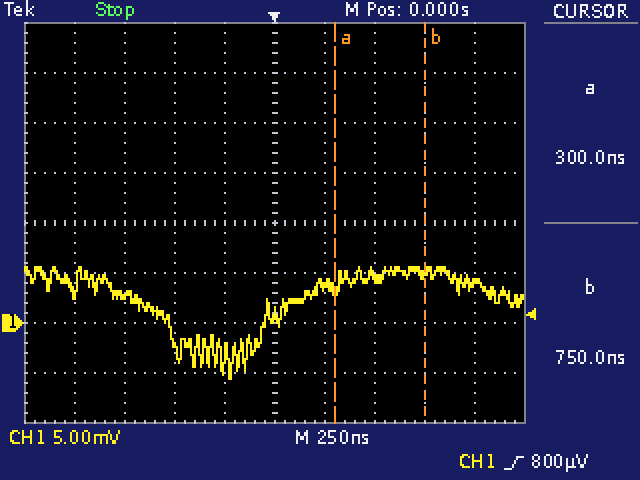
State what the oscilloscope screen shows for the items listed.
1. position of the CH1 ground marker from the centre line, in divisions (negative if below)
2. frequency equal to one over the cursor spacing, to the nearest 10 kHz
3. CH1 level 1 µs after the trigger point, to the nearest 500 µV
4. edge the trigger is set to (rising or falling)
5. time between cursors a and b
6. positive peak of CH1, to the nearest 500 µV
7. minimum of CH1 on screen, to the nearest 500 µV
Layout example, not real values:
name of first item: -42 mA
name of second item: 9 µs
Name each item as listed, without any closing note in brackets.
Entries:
position of the CH1 ground marker from the centre line, in divisions: -2.0 div
frequency equal to one over the cursor spacing, to the nearest 10 kHz: 2.22 MHz
CH1 level 1 µs after the trigger point, to the nearest 500 µV: 4.0 mV
edge the trigger is set to: rising
time between cursors a and b: 450 ns
positive peak of CH1, to the nearest 500 µV: 5.5 mV
minimum of CH1 on screen, to the nearest 500 µV: -5.5 mV
